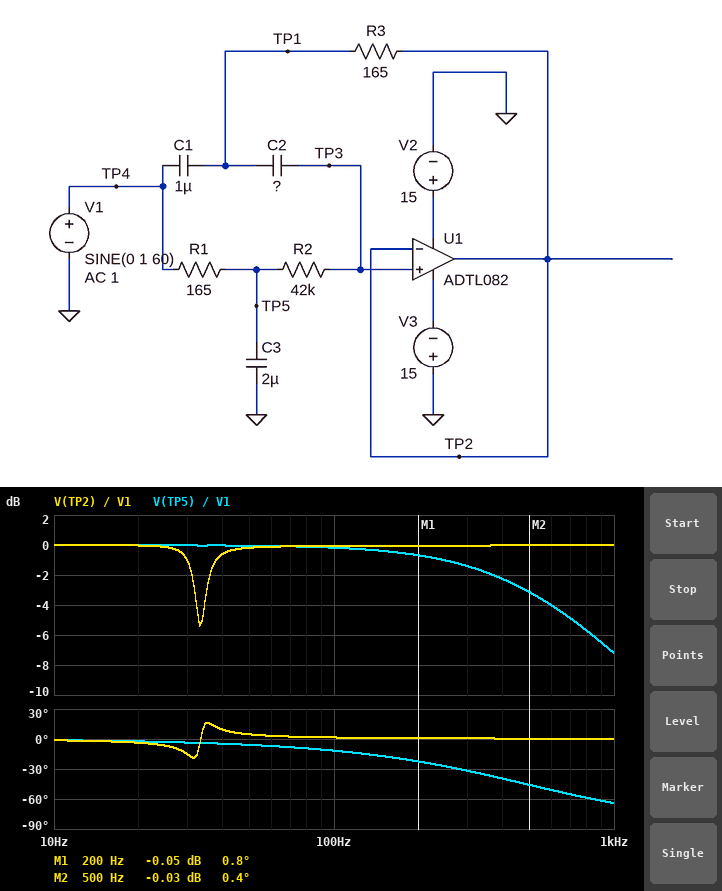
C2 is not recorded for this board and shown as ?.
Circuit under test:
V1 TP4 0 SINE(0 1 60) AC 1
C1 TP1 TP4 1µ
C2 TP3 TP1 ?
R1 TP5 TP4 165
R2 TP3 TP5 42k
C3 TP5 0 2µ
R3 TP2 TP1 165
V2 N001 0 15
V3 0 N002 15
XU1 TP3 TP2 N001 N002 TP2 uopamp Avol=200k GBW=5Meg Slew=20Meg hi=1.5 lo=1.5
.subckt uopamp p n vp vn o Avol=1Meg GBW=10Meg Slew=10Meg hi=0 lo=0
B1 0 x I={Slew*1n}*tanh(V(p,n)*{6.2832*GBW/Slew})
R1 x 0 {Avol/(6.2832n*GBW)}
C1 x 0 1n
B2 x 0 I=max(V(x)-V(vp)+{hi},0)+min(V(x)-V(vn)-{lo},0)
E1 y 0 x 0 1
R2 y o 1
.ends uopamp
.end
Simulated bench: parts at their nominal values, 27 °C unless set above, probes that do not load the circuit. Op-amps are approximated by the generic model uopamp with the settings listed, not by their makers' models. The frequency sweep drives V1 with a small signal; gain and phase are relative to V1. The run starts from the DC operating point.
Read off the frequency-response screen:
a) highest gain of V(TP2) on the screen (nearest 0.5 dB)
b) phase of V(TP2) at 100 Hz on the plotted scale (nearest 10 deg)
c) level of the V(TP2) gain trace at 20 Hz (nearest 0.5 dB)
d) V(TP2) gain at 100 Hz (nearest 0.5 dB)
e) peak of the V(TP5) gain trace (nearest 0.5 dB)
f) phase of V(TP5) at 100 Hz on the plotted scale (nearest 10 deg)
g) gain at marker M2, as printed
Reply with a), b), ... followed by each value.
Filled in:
a) 0 dB
b) 0 deg
c) 0 dB
d) 0 dB
e) 0 dB
f) -10 deg
g) -0.03 dB
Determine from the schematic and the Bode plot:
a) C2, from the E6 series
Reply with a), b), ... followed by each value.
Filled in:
a) 3.3 µF
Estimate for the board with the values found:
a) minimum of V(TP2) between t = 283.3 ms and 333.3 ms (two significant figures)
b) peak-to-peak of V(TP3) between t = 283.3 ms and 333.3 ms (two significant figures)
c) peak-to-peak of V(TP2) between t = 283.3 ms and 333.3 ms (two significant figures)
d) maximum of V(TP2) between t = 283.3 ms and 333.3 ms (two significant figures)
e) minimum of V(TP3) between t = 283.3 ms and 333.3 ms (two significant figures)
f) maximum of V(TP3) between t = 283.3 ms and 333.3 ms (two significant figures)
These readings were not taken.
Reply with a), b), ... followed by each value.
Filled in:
a) -990 mV
b) 2.0 V
c) 2.0 V
d) 990 mV
e) -990 mV
f) 990 mV
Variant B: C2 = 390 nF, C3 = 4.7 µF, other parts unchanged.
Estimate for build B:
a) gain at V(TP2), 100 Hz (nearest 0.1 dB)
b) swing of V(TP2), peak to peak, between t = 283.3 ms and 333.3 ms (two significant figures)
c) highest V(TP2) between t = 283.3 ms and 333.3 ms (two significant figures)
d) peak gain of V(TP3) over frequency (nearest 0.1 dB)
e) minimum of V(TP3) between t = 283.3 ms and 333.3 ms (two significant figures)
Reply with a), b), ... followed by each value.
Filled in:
a) 6.5 dB
b) 1.9 V
c) 950 mV
d) 6.7 dB
e) -950 mV
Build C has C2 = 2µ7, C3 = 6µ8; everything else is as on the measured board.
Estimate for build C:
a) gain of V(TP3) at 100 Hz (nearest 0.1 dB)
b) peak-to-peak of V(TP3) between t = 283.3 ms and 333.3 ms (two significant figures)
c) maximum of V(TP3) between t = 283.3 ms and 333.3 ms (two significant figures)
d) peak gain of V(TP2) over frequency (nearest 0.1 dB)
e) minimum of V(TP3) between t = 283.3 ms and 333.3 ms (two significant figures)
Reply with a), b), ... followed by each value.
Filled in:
a) 0.2 dB
b) 2.1 V
c) 1.0 V
d) 0.4 dB
e) -1.0 V
